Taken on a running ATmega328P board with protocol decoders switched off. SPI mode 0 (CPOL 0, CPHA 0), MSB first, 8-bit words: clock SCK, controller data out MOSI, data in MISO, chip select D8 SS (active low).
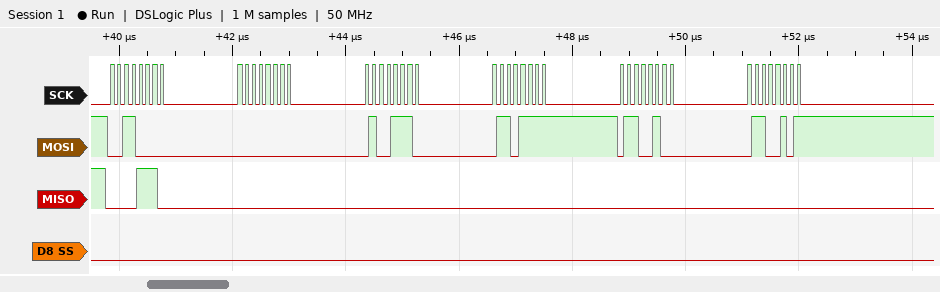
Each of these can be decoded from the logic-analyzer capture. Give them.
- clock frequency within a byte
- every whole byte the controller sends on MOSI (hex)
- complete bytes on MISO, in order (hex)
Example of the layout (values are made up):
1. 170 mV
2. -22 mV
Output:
1. 8 MHz
2. 30 00 4E 6F 64 65
3. 0E 00 00 00 00 00
